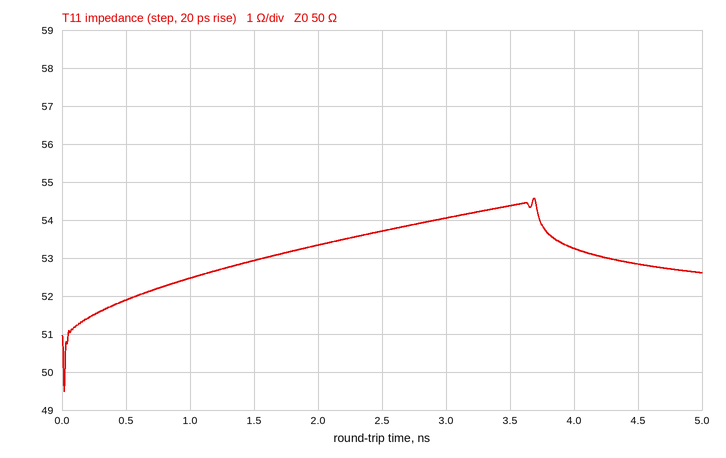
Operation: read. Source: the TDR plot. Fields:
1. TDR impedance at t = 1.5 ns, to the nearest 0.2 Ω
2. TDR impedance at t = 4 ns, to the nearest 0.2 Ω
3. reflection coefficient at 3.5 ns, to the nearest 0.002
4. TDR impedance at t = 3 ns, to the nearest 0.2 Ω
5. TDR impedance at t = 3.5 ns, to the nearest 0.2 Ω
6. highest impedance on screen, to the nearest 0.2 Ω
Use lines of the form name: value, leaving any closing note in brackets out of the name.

TDR impedance at t = 1.5 ns, to the nearest 0.2 Ω: 53.0 Ω
TDR impedance at t = 4 ns, to the nearest 0.2 Ω: 53.2 Ω
reflection coefficient at 3.5 ns, to the nearest 0.002: +0.042
TDR impedance at t = 3 ns, to the nearest 0.2 Ω: 54.0 Ω
TDR impedance at t = 3.5 ns, to the nearest 0.2 Ω: 54.4 Ω
highest impedance on screen, to the nearest 0.2 Ω: 54.6 Ω
